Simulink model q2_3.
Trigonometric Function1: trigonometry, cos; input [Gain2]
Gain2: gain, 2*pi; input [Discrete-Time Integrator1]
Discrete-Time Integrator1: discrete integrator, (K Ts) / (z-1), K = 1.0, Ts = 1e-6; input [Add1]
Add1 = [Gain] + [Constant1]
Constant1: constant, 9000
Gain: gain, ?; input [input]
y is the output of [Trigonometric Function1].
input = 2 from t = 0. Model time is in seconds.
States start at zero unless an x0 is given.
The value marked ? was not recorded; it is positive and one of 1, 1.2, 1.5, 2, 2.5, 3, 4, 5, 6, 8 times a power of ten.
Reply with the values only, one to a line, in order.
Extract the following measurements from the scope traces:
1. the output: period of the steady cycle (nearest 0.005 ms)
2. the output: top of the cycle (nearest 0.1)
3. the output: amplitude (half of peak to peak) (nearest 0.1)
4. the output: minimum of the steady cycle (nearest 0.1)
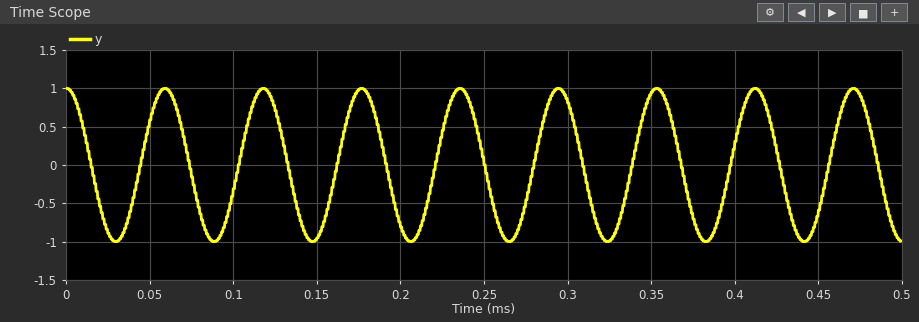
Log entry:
0.060 ms
1.0
1.0
-1.0
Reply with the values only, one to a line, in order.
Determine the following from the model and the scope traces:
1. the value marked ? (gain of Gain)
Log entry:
4000
